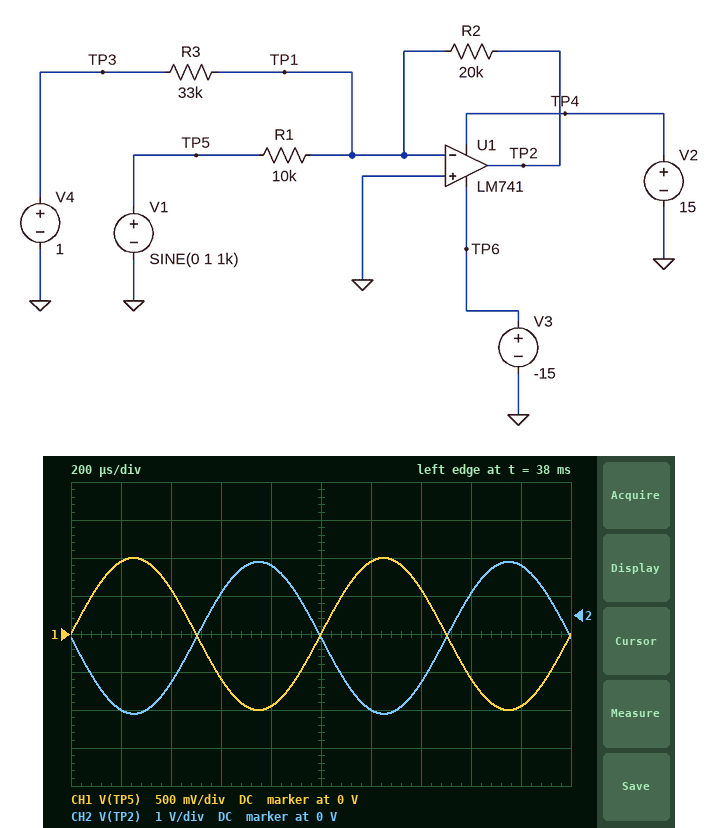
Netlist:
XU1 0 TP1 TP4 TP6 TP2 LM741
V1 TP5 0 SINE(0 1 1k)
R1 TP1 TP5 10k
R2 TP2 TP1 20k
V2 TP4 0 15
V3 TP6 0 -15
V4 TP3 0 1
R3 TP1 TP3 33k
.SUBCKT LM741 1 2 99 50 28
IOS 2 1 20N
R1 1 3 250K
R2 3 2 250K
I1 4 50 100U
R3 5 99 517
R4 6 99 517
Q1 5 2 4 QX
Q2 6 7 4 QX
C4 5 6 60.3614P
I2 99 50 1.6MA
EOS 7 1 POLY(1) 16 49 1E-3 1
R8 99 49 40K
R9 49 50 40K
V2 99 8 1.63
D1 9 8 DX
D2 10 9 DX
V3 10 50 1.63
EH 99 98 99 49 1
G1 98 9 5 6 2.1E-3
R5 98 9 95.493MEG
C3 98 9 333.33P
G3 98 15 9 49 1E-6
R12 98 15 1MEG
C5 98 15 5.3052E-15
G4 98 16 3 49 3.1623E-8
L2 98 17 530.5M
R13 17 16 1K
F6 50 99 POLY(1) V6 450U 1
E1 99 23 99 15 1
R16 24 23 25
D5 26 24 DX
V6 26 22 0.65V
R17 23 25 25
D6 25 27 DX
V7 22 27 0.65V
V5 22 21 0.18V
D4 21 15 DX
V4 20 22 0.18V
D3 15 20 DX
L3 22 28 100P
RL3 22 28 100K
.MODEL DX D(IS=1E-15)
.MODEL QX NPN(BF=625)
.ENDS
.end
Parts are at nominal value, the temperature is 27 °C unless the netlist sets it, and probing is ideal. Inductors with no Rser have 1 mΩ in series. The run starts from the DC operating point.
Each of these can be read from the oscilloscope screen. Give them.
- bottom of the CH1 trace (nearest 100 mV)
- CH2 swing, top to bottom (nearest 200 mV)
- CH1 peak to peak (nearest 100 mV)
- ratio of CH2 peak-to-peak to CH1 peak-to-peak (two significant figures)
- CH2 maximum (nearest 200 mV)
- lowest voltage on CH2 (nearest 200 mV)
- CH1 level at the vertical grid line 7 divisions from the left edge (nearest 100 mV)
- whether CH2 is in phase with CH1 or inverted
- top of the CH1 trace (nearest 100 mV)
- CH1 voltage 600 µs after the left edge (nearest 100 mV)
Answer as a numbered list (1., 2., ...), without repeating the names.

1. -1.0 V
2. 4.0 V
3. 2.0 V
4. 2.0
5. 1.4 V
6. -2.6 V
7. 600 mV
8. inverted
9. 1.0 V
10. -600 mV
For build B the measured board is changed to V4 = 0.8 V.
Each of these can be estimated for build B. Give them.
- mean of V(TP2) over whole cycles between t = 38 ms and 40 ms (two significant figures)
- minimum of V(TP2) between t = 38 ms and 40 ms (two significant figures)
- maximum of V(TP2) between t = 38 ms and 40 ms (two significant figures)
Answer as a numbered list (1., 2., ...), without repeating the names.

1. -480 mV
2. -2.5 V
3. 1.5 V
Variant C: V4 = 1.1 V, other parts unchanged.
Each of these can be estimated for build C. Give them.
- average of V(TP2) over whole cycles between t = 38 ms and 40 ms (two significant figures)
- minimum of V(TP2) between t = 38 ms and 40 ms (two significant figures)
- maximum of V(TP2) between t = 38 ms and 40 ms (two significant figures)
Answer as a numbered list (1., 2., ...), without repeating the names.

1. -660 mV
2. -2.7 V
3. 1.3 V
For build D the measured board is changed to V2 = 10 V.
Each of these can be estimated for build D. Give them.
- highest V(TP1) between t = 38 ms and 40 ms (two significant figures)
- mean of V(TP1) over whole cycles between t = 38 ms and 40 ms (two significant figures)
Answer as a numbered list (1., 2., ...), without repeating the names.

1. 3.1 mV
2. 1.1 mV
